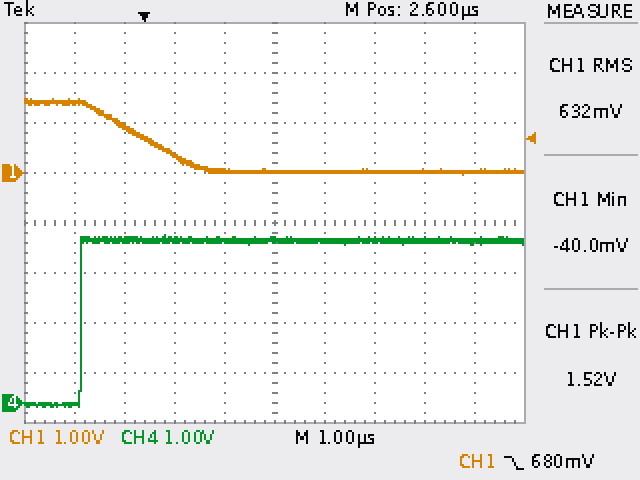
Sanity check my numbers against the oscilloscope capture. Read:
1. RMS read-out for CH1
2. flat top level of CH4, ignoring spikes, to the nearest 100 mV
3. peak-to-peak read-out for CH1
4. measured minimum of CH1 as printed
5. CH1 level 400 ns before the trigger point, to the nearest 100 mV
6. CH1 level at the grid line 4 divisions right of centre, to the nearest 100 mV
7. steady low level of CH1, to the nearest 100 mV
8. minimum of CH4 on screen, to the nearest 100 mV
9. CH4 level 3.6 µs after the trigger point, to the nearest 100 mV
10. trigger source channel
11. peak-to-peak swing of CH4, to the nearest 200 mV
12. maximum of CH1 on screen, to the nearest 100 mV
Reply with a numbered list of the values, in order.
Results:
1. 632 mV
2. 3.2 V
3. 1.52 V
4. -40.0 mV
5. 900 mV
6. 0.0 V
7. 0.0 V
8. -100 mV
9. 3.2 V
10. CH1
11. 3.4 V
12. 1.5 V
